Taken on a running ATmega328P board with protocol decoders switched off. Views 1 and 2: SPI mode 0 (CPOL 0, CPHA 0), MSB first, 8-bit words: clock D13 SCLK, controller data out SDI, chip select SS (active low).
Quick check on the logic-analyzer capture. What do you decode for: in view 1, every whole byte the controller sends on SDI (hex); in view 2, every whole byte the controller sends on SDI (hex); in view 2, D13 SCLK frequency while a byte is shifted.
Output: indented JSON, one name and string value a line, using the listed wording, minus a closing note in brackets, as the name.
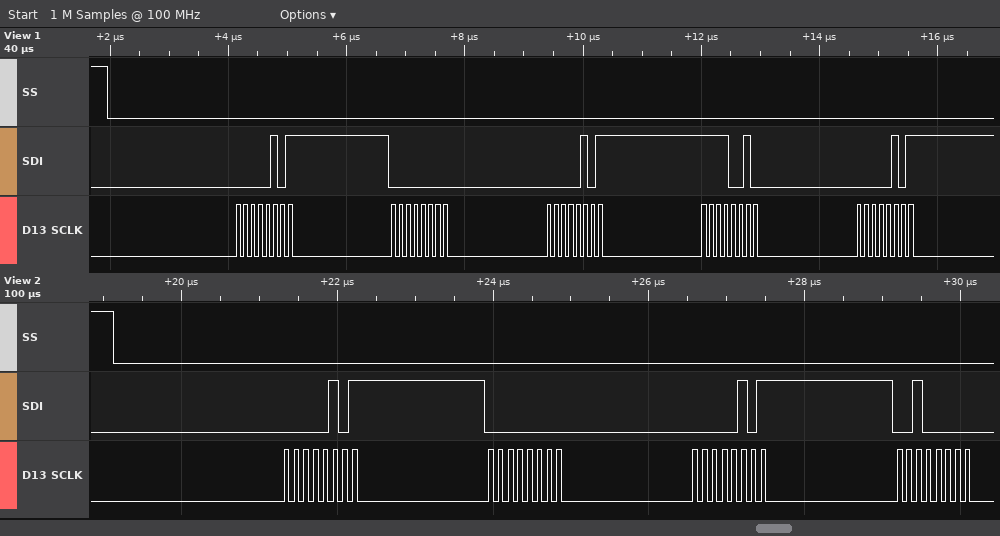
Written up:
{
  "in view 1, every whole byte the controller sends on SDI": "05 00 05 F2 05",
  "in view 2, every whole byte the controller sends on SDI": "05 00 05 20",
  "in view 2, D13 SCLK frequency while a byte is shifted": "8 MHz"
}
